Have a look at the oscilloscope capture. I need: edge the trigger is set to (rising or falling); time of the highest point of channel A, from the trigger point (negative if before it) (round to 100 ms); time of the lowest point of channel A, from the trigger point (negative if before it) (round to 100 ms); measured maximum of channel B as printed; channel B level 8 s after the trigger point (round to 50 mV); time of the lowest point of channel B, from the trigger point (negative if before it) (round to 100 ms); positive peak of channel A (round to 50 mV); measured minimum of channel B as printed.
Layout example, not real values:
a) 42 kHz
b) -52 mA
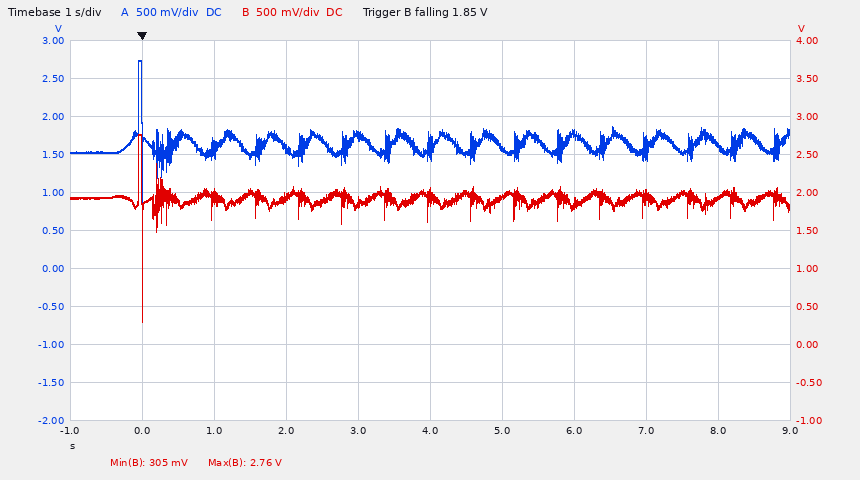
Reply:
a) falling
b) 0.0 s
c) 0.0 s
d) 2.76 V
e) 1.95 V
f) 0.0 s
g) 2.75 V
h) 305 mV
